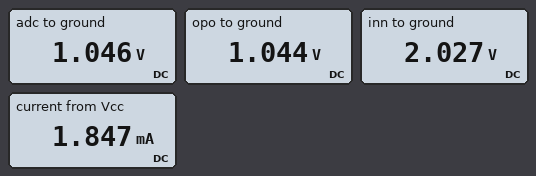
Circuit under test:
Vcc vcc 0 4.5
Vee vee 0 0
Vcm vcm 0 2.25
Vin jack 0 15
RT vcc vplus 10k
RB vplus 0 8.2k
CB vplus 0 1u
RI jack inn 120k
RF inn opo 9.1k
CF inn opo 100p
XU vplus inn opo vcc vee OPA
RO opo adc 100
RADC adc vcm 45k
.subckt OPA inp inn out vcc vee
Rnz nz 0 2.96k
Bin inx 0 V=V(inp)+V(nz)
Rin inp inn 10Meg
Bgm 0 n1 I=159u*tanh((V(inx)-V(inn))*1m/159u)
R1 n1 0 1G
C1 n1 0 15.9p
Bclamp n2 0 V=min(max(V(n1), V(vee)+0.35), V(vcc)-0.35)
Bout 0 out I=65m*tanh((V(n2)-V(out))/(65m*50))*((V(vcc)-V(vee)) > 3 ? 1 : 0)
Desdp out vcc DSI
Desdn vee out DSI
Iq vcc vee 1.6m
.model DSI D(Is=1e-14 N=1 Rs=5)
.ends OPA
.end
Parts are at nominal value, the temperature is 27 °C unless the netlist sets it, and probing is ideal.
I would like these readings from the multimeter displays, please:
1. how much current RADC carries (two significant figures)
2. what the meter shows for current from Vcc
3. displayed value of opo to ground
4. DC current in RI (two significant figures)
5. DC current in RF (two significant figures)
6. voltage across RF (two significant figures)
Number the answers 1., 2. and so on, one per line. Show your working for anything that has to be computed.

1. (2.25 V - 1.046 V) / 45 kΩ = 27 µA
2. 1.847 mA
3. 1.044 V
4. (15 V - 2.027 V) / 120 kΩ = 110 µA
5. (2.027 V - 1.044 V) / 9.1 kΩ = 110 µA
6. 2.027 V - 1.044 V = 980 mV
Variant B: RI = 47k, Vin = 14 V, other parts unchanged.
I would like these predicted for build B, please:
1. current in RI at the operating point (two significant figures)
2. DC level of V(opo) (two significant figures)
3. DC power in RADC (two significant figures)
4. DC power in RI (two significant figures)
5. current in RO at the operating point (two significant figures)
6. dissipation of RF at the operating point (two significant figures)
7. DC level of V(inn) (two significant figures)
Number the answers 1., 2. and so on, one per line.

1. 240 µA
2. 360 mV
3. 79 µW
4. 2.8 mW
5. 42 µA
6. 540 µW
7. 2.6 V
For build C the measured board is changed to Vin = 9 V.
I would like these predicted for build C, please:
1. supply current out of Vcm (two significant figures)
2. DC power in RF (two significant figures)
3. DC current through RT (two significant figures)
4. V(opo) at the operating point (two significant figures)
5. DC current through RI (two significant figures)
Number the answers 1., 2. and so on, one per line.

1. 17 µA
2. 31 µW
3. 250 µA
4. 1.5 V
5. 58 µA
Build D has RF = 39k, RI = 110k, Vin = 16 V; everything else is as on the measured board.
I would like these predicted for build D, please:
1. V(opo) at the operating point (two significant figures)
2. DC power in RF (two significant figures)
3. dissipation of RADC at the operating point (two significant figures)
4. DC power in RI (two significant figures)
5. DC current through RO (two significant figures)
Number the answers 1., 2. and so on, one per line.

1. 360 mV
2. 430 µW
3. 79 µW
4. 1.2 mW
5. 42 µA
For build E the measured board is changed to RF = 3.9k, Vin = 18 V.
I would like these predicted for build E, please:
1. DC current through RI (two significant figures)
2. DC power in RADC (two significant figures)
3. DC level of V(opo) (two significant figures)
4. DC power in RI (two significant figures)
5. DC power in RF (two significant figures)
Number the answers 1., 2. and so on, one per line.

1. 130 µA
2. 12 µW
3. 1.5 V
4. 2.1 mW
5. 69 µW
